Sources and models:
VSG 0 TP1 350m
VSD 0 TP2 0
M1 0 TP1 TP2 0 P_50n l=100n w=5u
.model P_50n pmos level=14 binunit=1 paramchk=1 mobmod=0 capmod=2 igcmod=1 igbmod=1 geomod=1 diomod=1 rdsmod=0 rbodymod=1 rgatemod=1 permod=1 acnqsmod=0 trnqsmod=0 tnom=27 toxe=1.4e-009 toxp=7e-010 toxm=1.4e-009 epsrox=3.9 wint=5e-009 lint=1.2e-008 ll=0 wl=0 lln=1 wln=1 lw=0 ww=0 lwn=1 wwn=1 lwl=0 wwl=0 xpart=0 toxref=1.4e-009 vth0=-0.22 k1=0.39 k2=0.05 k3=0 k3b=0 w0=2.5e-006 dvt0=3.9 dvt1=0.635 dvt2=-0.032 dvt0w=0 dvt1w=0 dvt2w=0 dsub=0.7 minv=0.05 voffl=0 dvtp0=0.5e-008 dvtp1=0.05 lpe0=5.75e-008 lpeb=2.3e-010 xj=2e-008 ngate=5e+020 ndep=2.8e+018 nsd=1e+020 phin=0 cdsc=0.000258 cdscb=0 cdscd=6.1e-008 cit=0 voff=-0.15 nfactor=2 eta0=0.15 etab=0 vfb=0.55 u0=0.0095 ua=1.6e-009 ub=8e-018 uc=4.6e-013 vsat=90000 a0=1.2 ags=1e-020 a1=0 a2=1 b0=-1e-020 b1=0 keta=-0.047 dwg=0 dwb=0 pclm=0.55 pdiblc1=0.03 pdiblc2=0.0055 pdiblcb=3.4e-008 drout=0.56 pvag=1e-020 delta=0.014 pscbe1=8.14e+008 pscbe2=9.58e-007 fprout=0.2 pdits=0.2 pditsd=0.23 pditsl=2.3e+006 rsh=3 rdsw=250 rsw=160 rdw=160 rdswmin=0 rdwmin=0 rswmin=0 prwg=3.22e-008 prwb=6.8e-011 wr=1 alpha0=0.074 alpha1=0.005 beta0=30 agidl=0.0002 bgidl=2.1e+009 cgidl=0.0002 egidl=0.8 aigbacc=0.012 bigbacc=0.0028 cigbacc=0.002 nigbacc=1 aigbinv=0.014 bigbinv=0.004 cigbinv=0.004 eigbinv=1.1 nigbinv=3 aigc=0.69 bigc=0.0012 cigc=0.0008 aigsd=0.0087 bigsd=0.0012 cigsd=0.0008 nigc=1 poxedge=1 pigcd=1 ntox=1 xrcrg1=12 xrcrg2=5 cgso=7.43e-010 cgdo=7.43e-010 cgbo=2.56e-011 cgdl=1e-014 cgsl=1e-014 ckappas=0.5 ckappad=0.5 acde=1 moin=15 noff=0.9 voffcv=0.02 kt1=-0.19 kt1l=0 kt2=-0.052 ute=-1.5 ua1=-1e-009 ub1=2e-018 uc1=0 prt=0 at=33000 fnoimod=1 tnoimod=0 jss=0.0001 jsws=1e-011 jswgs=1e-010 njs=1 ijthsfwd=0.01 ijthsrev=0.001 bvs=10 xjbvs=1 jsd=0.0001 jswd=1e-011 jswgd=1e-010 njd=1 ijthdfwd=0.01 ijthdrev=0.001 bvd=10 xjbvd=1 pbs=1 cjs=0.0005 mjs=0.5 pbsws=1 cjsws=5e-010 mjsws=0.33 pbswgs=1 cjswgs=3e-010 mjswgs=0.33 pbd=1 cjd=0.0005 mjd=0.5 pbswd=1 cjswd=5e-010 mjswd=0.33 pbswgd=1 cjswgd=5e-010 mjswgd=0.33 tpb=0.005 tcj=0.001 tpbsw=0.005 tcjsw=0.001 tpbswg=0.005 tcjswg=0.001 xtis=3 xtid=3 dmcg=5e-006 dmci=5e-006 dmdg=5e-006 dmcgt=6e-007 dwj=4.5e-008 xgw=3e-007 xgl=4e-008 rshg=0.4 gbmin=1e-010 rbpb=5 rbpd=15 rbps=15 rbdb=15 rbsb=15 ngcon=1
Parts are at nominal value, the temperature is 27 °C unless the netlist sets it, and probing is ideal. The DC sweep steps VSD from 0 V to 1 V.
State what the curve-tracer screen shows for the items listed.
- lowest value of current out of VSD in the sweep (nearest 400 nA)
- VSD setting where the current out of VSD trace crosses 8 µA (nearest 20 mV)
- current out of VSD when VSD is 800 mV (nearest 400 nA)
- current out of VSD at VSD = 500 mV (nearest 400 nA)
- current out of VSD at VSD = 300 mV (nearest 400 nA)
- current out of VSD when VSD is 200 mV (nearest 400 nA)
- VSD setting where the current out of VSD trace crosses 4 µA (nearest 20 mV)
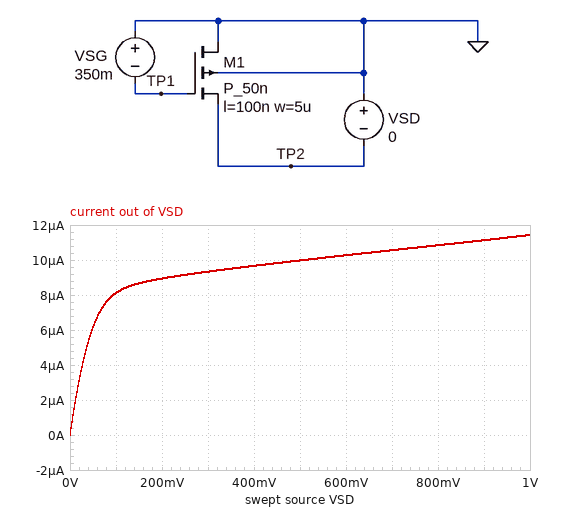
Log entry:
0 A
100 mV
10.8 µA
10.0 µA
9.2 µA
8.8 µA
20 mV
